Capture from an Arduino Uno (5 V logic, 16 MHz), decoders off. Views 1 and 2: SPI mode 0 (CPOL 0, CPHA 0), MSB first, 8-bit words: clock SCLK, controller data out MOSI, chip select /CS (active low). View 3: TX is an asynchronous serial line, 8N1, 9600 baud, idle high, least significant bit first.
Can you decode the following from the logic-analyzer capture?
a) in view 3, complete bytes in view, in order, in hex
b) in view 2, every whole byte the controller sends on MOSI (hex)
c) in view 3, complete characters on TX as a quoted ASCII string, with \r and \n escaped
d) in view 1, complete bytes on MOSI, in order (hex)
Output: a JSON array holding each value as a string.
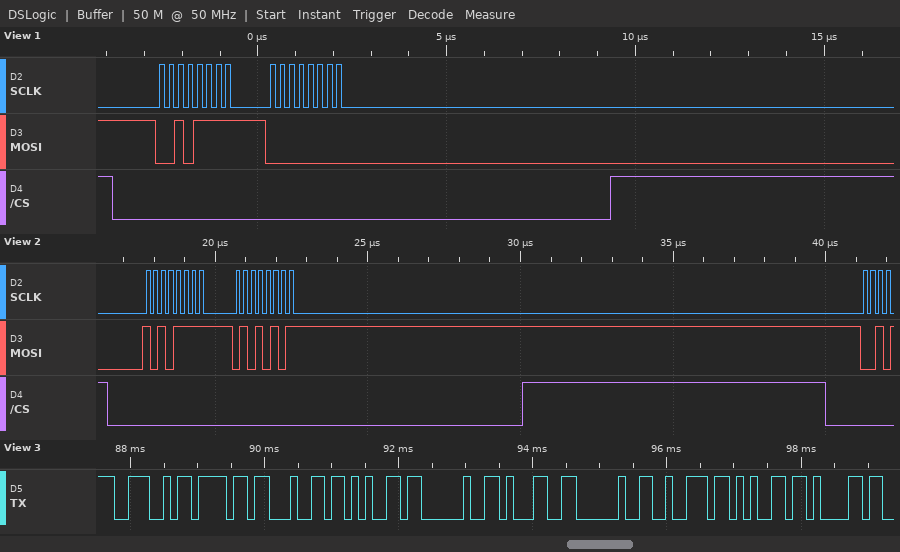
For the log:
["0x4E 0x6F 0x64 0x65 0x20 0x31 0x20 0x72 0x65 0x61", "AF 55", "\"Node 1 rea\"", "2F 00"]
